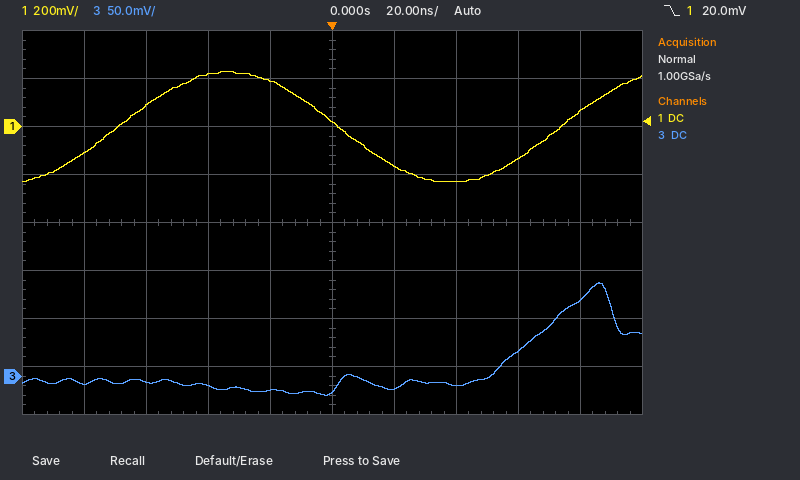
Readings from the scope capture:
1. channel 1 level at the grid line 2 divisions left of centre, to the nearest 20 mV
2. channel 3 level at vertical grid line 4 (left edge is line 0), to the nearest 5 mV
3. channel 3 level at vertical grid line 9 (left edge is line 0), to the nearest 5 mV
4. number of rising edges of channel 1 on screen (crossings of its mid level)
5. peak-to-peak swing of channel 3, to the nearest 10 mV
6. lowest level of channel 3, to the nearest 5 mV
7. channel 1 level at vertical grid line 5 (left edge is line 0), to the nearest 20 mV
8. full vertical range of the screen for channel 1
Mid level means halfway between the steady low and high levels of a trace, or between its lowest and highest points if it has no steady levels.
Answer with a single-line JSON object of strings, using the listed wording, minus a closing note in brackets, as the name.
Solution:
{"channel 1 level at the grid line 2 divisions left of centre, to the nearest 20 mV": "220 mV", "channel 3 level at vertical grid line 4 (left edge is line 0), to the nearest 5 mV": "-15 mV", "channel 3 level at vertical grid line 9 (left edge is line 0), to the nearest 5 mV": "80 mV", "number of rising edges of channel 1 on screen": "2", "peak-to-peak swing of channel 3, to the nearest 10 mV": "120 mV", "lowest level of channel 3, to the nearest 5 mV": "-20 mV", "channel 1 level at vertical grid line 5 (left edge is line 0), to the nearest 20 mV": "20 mV", "full vertical range of the screen for channel 1": "1.6 V"}
